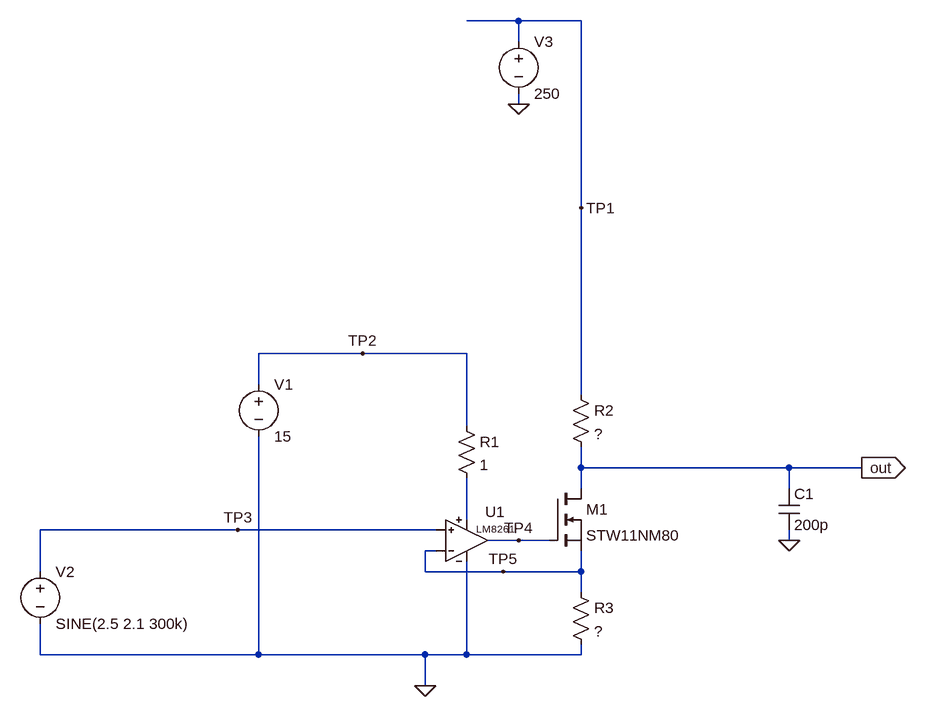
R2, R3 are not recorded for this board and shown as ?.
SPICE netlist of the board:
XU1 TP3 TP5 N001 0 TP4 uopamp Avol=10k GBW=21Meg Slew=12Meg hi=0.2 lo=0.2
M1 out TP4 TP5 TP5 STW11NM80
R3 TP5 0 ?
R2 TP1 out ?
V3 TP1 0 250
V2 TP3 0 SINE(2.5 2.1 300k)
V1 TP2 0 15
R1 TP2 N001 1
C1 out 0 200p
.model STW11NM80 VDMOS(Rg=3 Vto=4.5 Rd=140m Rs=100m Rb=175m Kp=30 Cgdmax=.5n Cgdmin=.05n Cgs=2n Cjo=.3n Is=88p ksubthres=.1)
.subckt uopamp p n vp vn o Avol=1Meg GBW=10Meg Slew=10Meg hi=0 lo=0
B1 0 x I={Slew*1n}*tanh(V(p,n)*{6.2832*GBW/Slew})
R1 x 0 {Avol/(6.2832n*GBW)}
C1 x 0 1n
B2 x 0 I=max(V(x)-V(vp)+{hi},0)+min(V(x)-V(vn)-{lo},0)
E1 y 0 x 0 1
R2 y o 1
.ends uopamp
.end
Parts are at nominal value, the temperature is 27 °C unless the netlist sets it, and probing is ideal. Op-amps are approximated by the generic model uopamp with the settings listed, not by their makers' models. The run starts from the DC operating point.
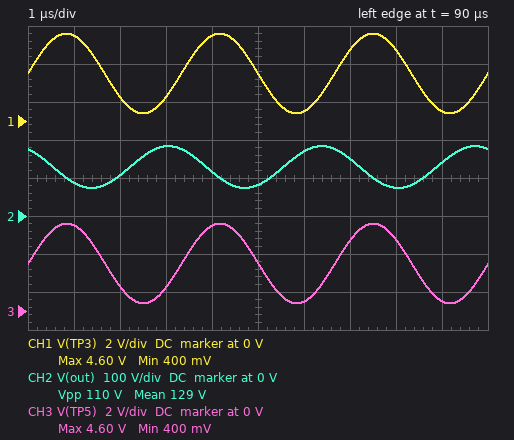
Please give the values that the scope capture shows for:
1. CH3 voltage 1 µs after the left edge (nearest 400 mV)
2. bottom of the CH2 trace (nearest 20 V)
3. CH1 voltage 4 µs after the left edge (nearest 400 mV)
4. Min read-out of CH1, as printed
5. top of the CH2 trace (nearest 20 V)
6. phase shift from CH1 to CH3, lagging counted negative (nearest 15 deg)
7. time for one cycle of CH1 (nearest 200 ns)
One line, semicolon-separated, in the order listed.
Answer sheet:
4.4 V; 80 V; 4.4 V; 400 mV; 180 V; 0 deg; 3.4 µs
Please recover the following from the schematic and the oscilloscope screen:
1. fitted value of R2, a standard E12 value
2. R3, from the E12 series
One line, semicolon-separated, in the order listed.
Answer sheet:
3.3 kΩ; 68 Ω
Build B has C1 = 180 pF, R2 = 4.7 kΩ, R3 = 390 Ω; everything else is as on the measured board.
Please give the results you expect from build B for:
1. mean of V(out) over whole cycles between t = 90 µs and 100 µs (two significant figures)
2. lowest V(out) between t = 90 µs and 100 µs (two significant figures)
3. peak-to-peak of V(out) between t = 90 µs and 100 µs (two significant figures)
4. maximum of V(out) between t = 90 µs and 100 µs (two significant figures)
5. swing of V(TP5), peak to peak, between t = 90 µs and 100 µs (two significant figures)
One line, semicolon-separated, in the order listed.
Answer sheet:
220 V; 210 V; 22 V; 230 V; 4.2 V
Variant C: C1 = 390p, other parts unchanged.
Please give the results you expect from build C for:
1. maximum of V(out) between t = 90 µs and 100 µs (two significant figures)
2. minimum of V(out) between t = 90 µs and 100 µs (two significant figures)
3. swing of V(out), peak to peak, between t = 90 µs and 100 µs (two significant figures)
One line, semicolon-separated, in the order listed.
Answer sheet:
160 V; 94 V; 70 V
